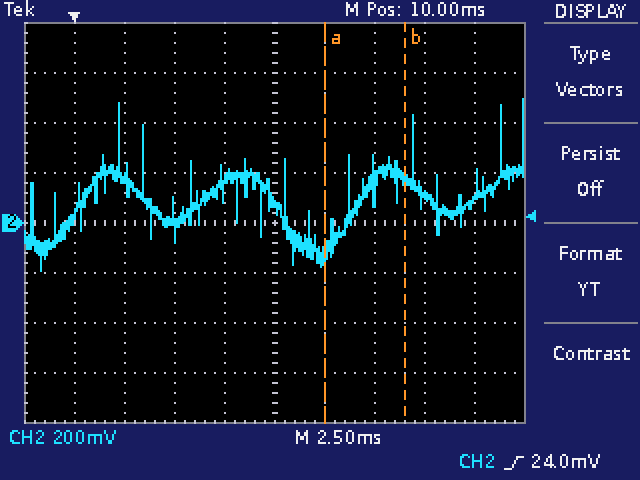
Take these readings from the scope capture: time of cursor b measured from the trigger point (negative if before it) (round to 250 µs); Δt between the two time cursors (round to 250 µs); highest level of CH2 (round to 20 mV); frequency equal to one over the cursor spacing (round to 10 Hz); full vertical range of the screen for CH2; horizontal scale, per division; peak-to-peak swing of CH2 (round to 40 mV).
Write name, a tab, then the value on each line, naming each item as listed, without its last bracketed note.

time of cursor b measured from the trigger point (negative if before it)	+16.50 ms
Δt between the two time cursors	4.00 ms
highest level of CH2	500 mV
frequency equal to one over the cursor spacing	250 Hz
full vertical range of the screen for CH2	1.6 V
horizontal scale, per division	2.5 ms
peak-to-peak swing of CH2	680 mV
